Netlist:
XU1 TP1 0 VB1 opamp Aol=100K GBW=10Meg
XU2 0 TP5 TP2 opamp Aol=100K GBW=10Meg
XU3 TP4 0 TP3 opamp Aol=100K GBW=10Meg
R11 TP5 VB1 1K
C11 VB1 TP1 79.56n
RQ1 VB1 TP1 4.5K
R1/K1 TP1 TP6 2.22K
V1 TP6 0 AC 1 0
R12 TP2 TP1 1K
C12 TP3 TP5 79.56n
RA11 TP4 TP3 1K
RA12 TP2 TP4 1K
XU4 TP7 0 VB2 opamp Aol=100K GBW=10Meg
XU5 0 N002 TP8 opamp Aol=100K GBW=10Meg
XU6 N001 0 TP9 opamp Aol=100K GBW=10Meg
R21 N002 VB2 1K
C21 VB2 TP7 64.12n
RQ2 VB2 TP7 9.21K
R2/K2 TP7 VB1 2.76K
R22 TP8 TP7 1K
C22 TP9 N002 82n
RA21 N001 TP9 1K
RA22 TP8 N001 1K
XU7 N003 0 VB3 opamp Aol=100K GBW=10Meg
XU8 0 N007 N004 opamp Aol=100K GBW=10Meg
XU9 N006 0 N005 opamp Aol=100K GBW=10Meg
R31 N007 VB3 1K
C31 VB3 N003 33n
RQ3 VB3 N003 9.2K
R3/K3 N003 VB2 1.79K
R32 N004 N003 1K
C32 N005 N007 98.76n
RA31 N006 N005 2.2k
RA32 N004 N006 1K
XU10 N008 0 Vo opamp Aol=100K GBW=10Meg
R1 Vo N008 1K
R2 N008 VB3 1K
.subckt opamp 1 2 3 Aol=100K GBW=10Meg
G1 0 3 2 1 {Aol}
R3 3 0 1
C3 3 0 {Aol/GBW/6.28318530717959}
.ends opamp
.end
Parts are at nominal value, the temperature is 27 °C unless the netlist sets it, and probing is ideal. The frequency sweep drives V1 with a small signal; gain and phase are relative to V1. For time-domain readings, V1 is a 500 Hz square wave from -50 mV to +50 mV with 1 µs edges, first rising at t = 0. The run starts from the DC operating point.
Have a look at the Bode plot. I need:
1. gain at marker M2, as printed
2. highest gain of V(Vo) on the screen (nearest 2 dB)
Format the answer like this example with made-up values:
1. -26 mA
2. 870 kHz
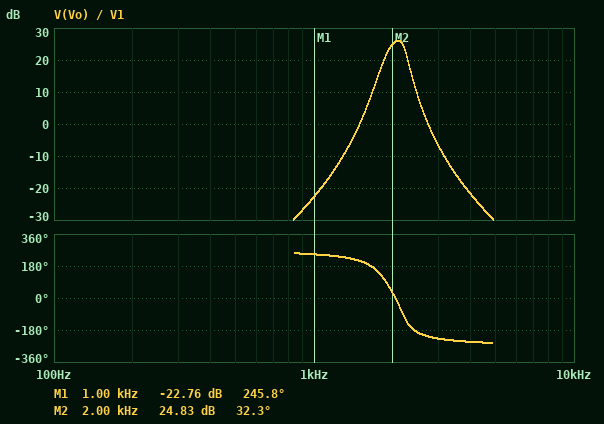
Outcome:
1. 24.83 dB
2. 26 dB
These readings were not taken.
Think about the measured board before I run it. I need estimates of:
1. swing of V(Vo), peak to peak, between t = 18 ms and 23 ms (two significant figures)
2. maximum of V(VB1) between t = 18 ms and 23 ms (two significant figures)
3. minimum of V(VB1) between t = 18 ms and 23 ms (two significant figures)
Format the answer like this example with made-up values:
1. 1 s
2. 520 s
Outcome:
1. 120 mV
2. 31 mV
3. -31 mV
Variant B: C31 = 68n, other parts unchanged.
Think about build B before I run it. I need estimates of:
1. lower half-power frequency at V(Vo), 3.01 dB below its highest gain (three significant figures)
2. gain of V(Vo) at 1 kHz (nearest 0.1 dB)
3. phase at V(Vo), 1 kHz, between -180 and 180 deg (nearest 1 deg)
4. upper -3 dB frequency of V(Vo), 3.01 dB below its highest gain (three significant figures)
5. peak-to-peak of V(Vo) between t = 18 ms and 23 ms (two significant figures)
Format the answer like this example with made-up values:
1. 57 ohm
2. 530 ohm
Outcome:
1. 1.95 kHz
2. -18.4 dB
3. -122 deg
4. 2.25 kHz
5. 67 mV
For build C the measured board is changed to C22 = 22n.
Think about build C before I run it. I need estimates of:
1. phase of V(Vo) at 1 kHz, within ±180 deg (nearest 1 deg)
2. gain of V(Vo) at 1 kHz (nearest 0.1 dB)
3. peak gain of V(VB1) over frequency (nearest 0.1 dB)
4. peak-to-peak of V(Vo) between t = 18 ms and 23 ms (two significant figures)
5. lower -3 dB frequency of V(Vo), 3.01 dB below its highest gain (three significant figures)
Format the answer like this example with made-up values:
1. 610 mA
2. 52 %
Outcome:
1. -111 deg
2. -35.7 dB
3. 6.1 dB
4. 19 mV
5. 1.82 kHz
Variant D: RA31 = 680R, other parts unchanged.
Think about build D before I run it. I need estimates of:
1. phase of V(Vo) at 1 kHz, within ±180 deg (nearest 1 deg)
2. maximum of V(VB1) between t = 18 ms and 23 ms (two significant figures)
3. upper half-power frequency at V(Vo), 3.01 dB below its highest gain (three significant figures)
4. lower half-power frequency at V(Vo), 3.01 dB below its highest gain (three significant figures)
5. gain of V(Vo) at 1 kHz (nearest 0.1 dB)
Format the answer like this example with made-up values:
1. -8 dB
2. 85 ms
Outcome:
1. -105 deg
2. 31 mV
3. 2.30 kHz
4. 2.04 kHz
5. -34.9 dB
